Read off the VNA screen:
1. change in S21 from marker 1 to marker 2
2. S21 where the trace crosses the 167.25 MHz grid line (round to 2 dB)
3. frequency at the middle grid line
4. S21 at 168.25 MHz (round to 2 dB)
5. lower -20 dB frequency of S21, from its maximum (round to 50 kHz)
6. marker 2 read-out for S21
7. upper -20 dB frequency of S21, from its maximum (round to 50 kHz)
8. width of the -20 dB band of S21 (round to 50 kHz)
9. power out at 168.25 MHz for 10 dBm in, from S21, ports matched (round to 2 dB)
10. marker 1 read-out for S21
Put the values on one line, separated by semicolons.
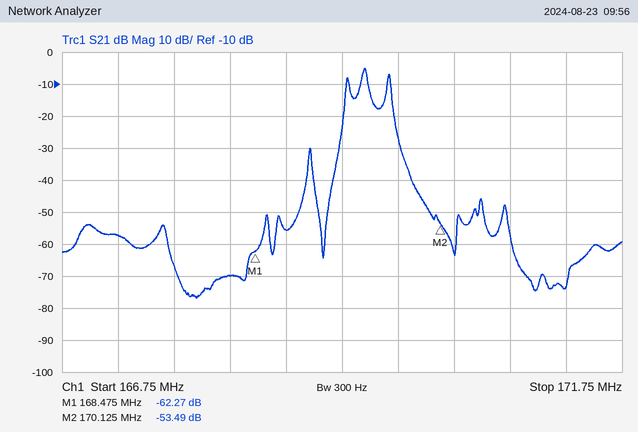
8.78 dB; -58 dB; 169.25 MHz; -70 dB; 169.25 MHz; -53.49 dB; 169.75 MHz; 500 kHz; -60 dBm; -62.27 dB
